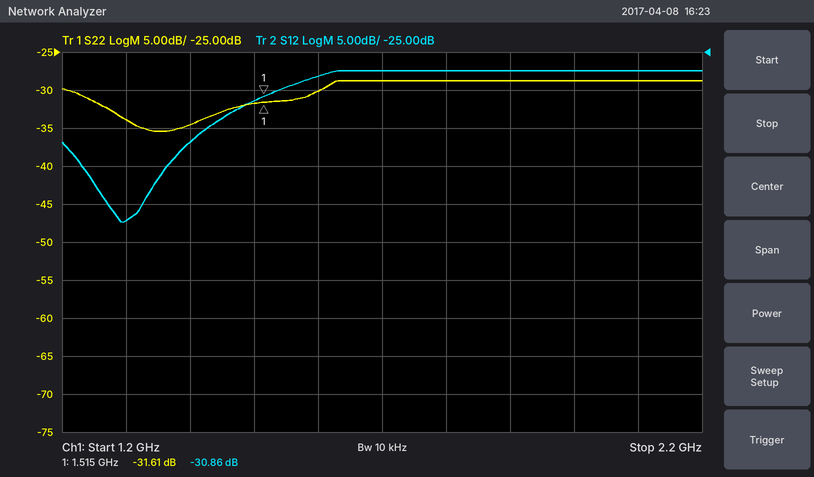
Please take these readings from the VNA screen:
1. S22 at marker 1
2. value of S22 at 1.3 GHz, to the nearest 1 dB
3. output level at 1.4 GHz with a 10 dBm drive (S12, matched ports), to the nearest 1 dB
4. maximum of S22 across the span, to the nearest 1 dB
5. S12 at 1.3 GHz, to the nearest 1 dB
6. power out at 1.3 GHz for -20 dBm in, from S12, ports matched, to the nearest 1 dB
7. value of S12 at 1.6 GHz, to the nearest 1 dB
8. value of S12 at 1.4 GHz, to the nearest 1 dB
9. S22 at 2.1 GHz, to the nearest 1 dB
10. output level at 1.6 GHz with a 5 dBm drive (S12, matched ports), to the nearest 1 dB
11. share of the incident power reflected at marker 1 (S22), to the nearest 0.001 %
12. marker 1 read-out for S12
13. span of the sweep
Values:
-31.61 dB
-34 dB
-27 dBm
-29 dB
-47 dB
-67 dBm
-28 dB
-37 dB
-29 dB
-23 dBm
0.069 %
-30.86 dB
1 GHz
